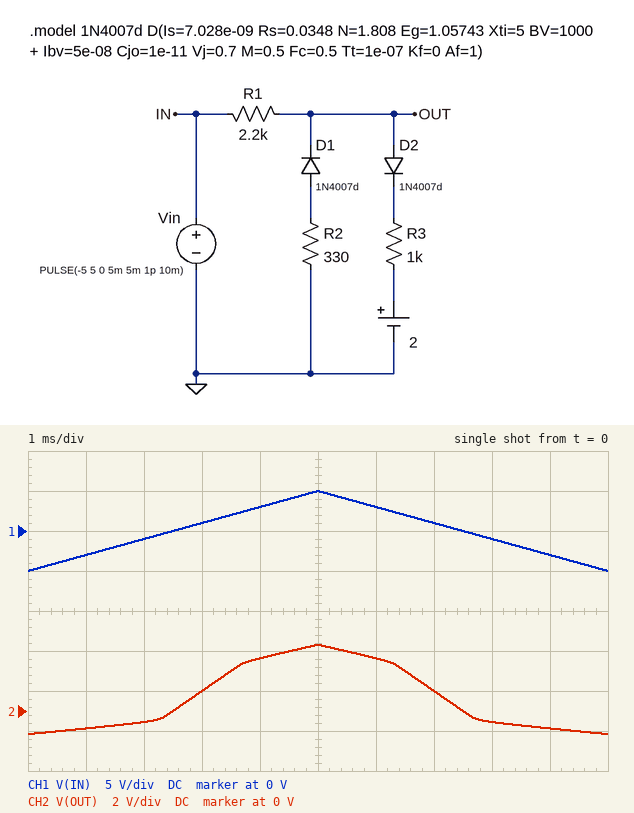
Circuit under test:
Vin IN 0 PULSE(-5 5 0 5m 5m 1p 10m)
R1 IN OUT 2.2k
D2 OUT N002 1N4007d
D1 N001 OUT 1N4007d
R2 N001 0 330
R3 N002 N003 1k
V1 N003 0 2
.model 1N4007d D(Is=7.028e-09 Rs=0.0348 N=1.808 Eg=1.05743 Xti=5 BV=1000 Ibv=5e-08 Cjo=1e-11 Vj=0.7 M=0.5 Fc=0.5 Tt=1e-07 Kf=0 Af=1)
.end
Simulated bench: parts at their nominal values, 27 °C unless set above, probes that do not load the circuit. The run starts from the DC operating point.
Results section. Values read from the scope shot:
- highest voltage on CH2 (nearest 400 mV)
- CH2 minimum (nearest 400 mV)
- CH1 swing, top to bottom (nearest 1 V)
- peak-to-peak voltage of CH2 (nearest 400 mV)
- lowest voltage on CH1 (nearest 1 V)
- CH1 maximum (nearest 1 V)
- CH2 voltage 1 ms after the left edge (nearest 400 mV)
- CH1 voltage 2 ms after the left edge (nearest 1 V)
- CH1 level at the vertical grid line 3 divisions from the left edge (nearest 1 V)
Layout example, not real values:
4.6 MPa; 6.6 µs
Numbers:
3.2 V; -1.2 V; 10 V; 4.4 V; -5 V; 5 V; -800 mV; -1 V; 1 V
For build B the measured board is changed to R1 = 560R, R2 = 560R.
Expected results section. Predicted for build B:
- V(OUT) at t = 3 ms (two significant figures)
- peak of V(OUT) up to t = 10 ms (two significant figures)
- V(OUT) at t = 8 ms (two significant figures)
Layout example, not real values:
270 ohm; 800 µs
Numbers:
1.0 V; 4.1 V; -760 mV
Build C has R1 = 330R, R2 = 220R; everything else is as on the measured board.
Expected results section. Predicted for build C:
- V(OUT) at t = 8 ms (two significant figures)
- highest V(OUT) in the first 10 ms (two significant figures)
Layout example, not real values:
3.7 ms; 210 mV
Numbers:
-730 mV; 4.4 V
